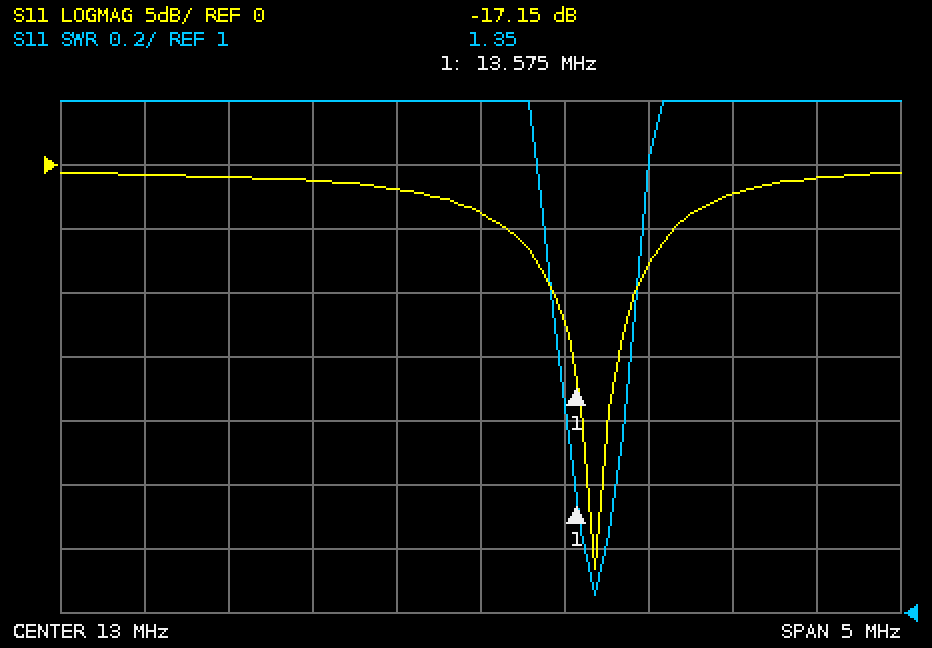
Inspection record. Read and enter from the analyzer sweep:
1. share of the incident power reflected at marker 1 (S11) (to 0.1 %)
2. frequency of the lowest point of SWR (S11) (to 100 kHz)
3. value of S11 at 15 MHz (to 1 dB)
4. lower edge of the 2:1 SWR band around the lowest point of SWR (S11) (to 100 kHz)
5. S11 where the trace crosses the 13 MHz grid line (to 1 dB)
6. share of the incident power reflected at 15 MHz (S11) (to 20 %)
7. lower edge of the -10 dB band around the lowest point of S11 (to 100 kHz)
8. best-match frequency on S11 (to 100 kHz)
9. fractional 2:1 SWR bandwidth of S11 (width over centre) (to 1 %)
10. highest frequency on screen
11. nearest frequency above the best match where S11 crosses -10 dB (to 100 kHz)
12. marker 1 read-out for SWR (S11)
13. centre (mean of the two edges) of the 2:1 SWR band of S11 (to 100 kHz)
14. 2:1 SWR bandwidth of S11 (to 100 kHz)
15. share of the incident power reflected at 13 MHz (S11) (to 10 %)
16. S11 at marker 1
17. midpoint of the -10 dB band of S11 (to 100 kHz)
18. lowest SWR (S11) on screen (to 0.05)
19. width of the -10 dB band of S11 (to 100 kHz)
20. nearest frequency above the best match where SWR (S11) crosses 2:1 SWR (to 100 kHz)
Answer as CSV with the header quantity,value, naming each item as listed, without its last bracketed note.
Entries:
quantity,value
share of the incident power reflected at marker 1 (S11),1.9 %
frequency of the lowest point of SWR (S11),13.7 MHz
value of S11 at 15 MHz,-1 dB
lower edge of the 2:1 SWR band around the lowest point of SWR (S11),13.4 MHz
S11 where the trace crosses the 13 MHz grid line,-4 dB
share of the incident power reflected at 15 MHz (S11),80 %
lower edge of the -10 dB band around the lowest point of S11,13.4 MHz
best-match frequency on S11,13.7 MHz
fractional 2:1 SWR bandwidth of S11 (width over centre),4 %
highest frequency on screen,15.5 MHz
nearest frequency above the best match where S11 crosses -10 dB,13.9 MHz
marker 1 read-out for SWR,1.35
centre (mean of the two edges) of the 2:1 SWR band of S11,13.7 MHz
2:1 SWR bandwidth of S11,500 kHz
share of the incident power reflected at 13 MHz (S11),40 %
S11 at marker 1,-17.15 dB
midpoint of the -10 dB band of S11,13.7 MHz
lowest SWR (S11) on screen,1.05
width of the -10 dB band of S11,500 kHz
nearest frequency above the best match where SWR (S11) crosses 2:1 SWR,13.9 MHz
